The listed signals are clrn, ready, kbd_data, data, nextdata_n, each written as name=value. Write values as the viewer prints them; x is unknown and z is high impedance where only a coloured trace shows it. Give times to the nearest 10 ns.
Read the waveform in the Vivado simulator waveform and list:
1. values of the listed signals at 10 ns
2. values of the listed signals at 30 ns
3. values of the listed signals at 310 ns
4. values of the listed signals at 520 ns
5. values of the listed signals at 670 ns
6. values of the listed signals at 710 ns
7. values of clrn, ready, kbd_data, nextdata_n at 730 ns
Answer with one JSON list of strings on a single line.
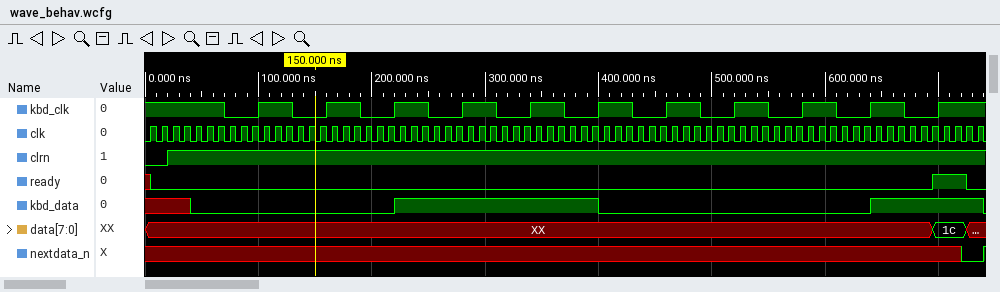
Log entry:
["clrn=0, ready=0, kbd_data=x, data=XX, nextdata_n=x", "clrn=1, ready=0, kbd_data=x, data=XX, nextdata_n=x", "clrn=1, ready=0, kbd_data=1, data=XX, nextdata_n=x", "clrn=1, ready=0, kbd_data=0, data=XX, nextdata_n=x", "clrn=1, ready=0, kbd_data=1, data=XX, nextdata_n=x", "clrn=1, ready=1, kbd_data=1, data=1c, nextdata_n=x", "clrn=1, ready=0, kbd_data=1, nextdata_n=0"]
